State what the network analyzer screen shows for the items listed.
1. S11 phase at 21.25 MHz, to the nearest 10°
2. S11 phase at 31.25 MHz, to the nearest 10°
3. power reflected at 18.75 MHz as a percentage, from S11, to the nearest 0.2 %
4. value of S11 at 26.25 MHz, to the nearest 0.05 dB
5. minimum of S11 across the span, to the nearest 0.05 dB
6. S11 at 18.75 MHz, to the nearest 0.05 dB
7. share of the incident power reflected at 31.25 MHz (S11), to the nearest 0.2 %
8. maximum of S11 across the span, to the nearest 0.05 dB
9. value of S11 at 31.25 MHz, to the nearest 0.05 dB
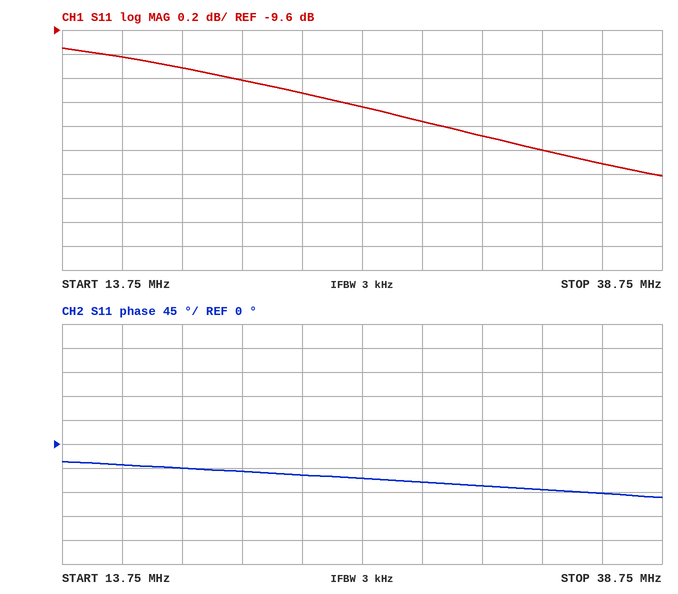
-50°
-80°
10.2 %
-10.25 dB
-10.80 dB
-9.90 dB
9.0 %
-9.75 dB
-10.50 dB
